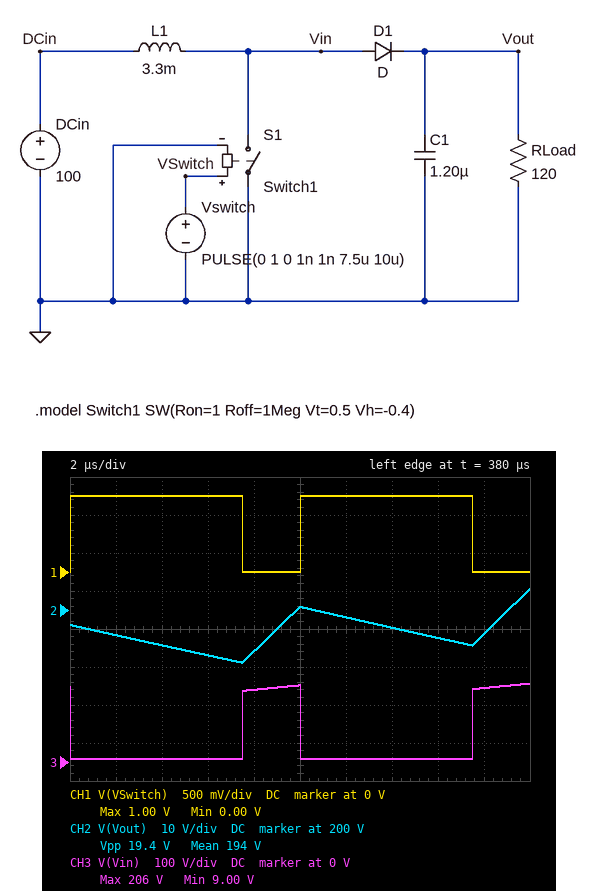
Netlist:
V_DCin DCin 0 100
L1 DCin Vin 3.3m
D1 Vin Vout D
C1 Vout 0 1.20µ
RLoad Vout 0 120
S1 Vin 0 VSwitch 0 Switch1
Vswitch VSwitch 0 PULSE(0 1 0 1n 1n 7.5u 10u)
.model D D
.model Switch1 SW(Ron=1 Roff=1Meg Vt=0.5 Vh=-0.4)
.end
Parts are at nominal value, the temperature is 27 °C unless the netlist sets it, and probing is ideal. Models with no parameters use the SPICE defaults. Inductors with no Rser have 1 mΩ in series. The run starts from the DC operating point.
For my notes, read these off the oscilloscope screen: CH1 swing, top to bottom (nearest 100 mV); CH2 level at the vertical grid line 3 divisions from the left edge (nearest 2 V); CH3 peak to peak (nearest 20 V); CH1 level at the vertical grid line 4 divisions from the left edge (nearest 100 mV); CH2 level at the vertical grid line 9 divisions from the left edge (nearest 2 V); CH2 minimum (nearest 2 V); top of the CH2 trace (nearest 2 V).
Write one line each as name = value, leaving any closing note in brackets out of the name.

CH1 swing, top to bottom = 1.0 V
CH2 level at the vertical grid line 3 divisions from the left edge = 188 V
CH3 peak to peak = 200 V
CH1 level at the vertical grid line 4 divisions from the left edge = 0 V
CH2 level at the vertical grid line 9 divisions from the left edge = 194 V
CH2 minimum = 186 V
top of the CH2 trace = 206 V
